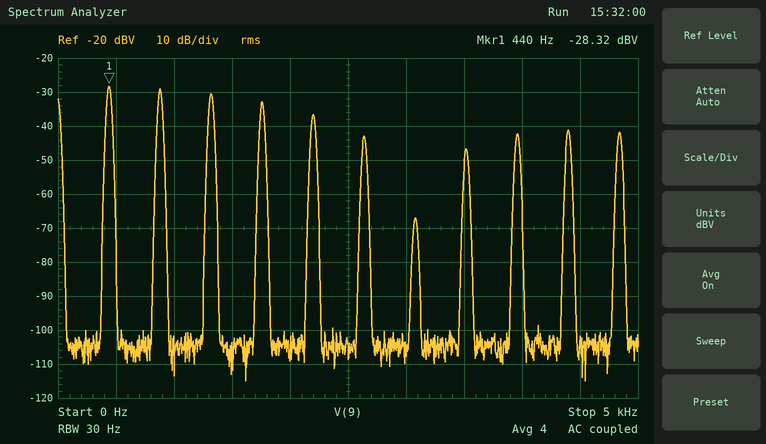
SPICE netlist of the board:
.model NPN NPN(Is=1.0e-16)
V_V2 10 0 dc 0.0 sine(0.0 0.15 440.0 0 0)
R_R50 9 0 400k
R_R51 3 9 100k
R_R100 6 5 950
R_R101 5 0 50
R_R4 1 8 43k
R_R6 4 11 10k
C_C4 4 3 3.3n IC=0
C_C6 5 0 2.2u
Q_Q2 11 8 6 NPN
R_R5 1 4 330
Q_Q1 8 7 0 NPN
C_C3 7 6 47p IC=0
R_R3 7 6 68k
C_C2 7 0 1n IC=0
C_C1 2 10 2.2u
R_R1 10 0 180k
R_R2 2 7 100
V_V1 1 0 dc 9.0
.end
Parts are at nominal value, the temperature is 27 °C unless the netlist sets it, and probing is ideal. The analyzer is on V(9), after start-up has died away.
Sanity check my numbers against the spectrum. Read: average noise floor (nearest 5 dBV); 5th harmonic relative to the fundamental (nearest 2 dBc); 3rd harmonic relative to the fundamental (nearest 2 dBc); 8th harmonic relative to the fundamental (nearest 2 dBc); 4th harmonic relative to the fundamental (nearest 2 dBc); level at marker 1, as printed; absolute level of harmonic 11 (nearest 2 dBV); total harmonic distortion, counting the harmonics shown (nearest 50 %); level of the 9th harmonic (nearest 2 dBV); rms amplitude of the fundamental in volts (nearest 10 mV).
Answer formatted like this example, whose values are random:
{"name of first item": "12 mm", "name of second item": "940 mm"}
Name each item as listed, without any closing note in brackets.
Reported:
{"average noise floor": "-105 dBV", "5th harmonic relative to the fundamental": "-8 dBc", "3rd harmonic relative to the fundamental": "-2 dBc", "8th harmonic relative to the fundamental": "-18 dBc", "4th harmonic relative to the fundamental": "-4 dBc", "level at marker 1, as printed": "-28.32 dBV", "absolute level of harmonic 11": "-42 dBV", "total harmonic distortion, counting the harmonics shown": "150 %", "level of the 9th harmonic": "-42 dBV", "rms amplitude of the fundamental in volts": "40 mV"}
